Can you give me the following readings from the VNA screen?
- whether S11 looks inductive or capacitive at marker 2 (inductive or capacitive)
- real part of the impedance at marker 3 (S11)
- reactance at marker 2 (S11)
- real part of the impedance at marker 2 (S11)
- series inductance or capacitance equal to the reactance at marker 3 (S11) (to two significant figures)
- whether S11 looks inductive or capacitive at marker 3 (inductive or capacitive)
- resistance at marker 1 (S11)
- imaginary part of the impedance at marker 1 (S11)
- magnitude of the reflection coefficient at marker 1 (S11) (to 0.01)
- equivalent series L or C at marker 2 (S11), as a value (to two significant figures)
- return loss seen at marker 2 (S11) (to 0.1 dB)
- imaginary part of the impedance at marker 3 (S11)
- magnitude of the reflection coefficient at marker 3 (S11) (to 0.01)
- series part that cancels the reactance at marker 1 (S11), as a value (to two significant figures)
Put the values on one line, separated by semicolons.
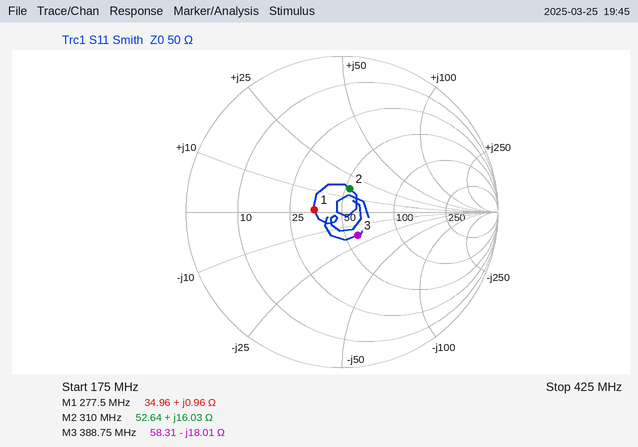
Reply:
inductive; 58.31 Ω; +16.03 Ω; 52.64 Ω; 23 pF; capacitive; 34.96 Ω; +0.96 Ω; 0.18; 8.2 nH; 16.1 dB; -18.01 Ω; 0.18; 600 pF
